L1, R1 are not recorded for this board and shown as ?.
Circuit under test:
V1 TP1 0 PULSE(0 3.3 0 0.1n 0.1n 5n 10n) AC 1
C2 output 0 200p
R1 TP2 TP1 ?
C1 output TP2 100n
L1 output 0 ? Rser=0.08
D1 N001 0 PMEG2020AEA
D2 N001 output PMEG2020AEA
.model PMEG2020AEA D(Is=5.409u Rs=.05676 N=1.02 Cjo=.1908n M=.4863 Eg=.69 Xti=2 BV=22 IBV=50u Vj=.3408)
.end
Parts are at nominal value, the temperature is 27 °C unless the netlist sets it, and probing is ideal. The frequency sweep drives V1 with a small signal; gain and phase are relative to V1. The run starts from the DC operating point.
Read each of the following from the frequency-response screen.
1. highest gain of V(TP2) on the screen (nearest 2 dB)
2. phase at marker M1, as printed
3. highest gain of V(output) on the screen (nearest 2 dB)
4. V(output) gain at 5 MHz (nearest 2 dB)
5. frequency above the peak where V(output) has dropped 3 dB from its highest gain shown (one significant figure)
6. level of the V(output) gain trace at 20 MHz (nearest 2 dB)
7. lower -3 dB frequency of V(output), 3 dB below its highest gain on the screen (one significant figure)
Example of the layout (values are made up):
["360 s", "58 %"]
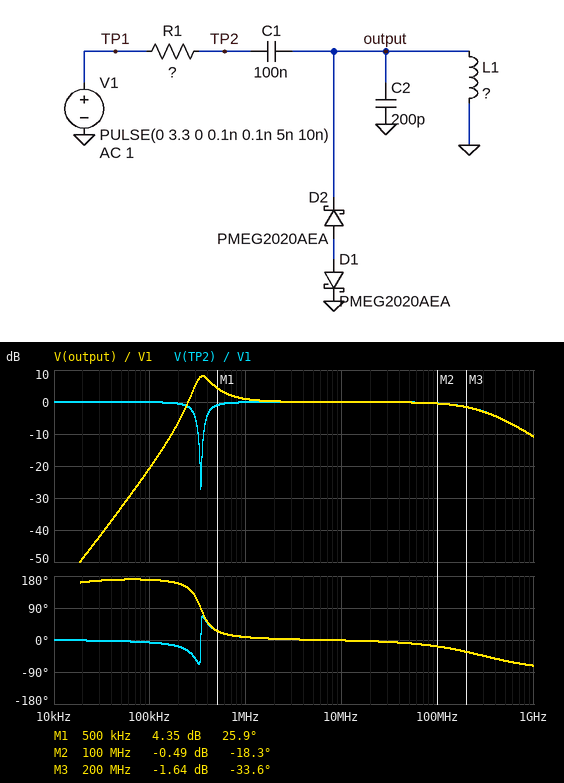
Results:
["0 dB", "25.9 deg", "8 dB", "0 dB", "500 kHz", "0 dB", "300 kHz"]
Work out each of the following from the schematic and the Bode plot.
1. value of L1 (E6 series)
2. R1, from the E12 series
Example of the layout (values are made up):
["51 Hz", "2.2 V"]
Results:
["2.2 µH", "1.8 Ω"]
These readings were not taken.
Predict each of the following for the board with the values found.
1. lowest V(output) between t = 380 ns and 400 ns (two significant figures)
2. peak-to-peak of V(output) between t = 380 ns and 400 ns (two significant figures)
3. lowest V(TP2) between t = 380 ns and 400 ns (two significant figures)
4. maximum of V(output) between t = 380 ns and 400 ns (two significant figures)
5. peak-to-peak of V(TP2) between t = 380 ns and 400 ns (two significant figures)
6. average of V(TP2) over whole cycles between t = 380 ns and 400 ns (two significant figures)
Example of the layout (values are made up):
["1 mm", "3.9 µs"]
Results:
["-930 mV", "3.3 V", "-410 mV", "2.4 V", "3.3 V", "1.3 V"]
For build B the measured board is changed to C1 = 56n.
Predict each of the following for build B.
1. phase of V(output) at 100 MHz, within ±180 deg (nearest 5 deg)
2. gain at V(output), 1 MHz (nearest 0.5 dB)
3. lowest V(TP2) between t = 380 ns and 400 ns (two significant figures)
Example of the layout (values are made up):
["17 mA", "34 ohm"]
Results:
["-20 deg", "2.0 dB", "-370 mV"]
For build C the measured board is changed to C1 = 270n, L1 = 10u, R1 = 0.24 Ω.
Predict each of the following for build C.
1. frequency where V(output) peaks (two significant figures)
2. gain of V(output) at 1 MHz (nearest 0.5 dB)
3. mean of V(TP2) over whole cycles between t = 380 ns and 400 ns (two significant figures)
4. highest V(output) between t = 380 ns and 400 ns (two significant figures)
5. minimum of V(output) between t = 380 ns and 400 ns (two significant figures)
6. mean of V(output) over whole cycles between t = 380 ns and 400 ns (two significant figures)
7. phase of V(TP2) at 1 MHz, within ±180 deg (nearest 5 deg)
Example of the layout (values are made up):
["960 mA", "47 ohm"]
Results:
["97 kHz", "0 dB", "1.7 V", "3.2 V", "-66 mV", "1.6 V", "0 deg"]
